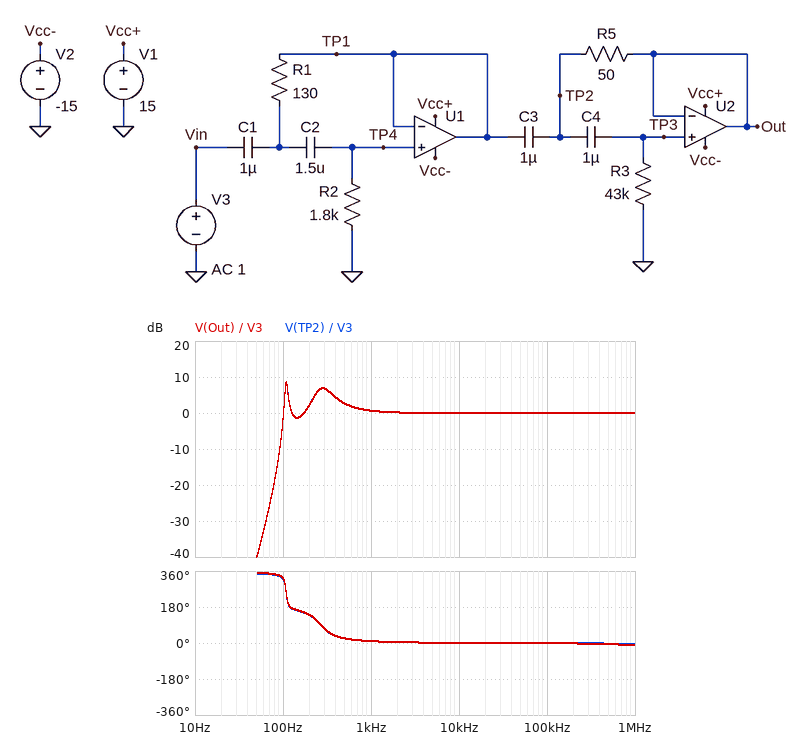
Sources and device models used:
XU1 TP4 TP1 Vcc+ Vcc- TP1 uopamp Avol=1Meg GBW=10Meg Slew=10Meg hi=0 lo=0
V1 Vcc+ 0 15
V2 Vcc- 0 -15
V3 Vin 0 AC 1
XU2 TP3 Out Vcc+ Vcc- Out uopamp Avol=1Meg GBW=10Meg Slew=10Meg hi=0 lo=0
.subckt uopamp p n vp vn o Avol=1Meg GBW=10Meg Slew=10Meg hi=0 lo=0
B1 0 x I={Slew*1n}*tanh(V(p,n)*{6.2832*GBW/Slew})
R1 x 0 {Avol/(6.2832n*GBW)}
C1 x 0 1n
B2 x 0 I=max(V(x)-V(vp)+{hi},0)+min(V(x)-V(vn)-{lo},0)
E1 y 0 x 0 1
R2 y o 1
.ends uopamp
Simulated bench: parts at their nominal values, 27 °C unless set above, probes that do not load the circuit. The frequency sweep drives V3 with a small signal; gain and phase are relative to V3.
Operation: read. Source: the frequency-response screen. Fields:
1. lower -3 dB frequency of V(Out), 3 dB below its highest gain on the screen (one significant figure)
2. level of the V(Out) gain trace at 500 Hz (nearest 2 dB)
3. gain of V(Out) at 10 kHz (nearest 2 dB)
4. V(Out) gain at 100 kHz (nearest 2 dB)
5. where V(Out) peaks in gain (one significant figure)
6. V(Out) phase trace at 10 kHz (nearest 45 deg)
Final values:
100 Hz
2 dB
0 dB
0 dB
100 Hz
0 deg
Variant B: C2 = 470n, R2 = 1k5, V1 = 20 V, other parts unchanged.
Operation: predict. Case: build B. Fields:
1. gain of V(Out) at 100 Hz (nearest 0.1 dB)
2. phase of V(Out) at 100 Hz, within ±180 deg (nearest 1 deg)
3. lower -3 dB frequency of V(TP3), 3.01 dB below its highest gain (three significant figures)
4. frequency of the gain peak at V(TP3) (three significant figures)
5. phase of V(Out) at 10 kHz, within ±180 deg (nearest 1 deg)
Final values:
-14.3 dB
-30 deg
439 Hz
582 Hz
2 deg
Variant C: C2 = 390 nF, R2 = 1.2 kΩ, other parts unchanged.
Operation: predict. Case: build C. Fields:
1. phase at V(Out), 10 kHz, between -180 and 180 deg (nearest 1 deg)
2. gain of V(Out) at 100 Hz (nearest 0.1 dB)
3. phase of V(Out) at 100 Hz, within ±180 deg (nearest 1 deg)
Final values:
3 deg
-17.9 dB
-29 deg
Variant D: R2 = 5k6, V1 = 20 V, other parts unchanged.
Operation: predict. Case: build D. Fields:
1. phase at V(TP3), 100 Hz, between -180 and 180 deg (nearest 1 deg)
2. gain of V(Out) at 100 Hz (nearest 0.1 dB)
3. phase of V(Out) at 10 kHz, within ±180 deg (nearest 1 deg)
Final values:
-42 deg
11.4 dB
0 deg
